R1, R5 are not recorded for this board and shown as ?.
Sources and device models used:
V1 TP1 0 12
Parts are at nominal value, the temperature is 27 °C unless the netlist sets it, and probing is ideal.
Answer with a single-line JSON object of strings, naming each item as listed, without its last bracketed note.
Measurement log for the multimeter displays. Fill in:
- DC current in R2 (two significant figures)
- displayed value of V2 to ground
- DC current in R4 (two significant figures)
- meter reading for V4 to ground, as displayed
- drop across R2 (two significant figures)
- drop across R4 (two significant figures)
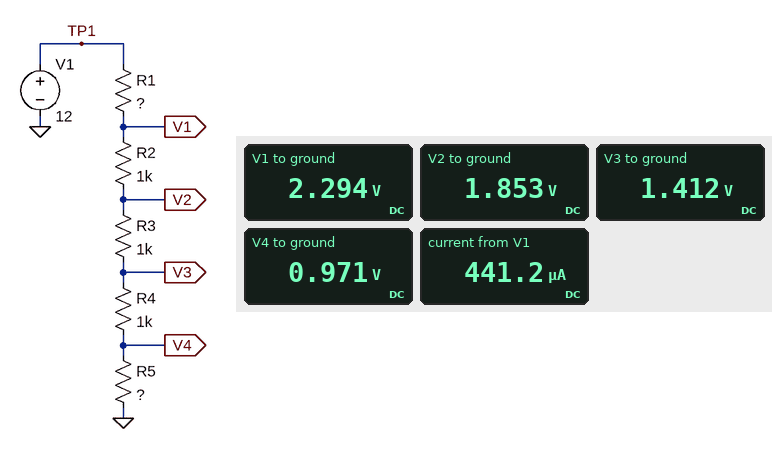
{"DC current in R2": "440 µA", "displayed value of V2 to ground": "1.853 V", "DC current in R4": "440 µA", "meter reading for V4 to ground, as displayed": "0.971 V", "drop across R2": "440 mV", "drop across R4": "440 mV"}
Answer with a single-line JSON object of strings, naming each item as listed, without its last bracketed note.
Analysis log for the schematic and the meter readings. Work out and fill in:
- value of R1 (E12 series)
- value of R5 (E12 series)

{"value of R1": "22 kΩ", "value of R5": "2.2 kΩ"}
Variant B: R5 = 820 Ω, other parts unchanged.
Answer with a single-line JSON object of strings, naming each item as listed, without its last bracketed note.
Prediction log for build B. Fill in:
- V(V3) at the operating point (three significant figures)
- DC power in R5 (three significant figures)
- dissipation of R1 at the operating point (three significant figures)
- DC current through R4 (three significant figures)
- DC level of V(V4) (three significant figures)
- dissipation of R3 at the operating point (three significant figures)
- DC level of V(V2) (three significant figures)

{"V(V3) at the operating point": "846 mV", "DC power in R5": "177 µW", "dissipation of R1 at the operating point": "4.75 mW", "DC current through R4": "465 µA", "DC level of V(V4)": "381 mV", "dissipation of R3 at the operating point": "216 µW", "DC level of V(V2)": "1.31 V"}
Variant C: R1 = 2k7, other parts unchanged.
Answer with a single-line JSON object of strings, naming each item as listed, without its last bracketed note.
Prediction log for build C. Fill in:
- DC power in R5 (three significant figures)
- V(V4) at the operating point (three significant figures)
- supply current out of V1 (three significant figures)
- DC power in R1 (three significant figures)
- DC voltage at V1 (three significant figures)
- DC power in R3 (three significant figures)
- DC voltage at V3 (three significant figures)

{"DC power in R5": "5.08 mW", "V(V4) at the operating point": "3.34 V", "supply current out of V1": "1.52 mA", "DC power in R1": "6.23 mW", "DC voltage at V1": "7.90 V", "DC power in R3": "2.31 mW", "DC voltage at V3": "4.86 V"}
